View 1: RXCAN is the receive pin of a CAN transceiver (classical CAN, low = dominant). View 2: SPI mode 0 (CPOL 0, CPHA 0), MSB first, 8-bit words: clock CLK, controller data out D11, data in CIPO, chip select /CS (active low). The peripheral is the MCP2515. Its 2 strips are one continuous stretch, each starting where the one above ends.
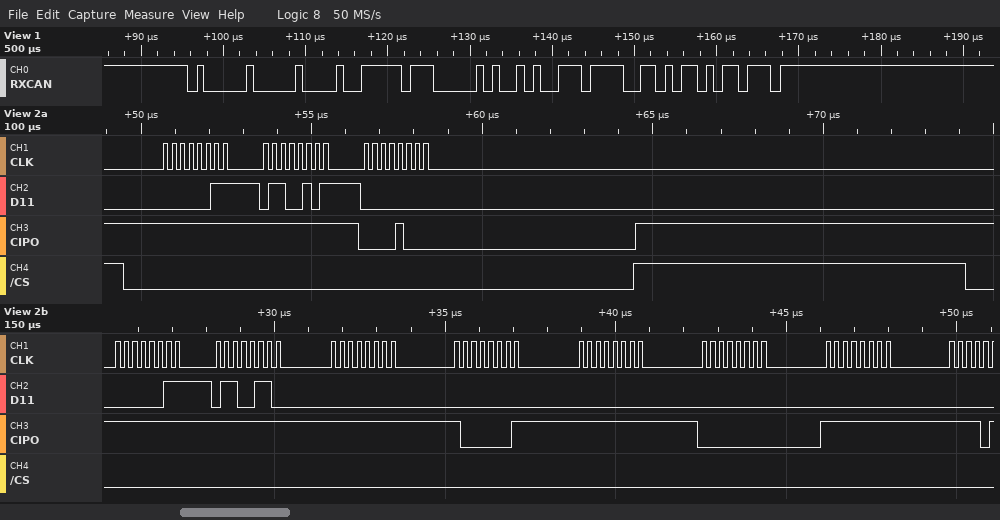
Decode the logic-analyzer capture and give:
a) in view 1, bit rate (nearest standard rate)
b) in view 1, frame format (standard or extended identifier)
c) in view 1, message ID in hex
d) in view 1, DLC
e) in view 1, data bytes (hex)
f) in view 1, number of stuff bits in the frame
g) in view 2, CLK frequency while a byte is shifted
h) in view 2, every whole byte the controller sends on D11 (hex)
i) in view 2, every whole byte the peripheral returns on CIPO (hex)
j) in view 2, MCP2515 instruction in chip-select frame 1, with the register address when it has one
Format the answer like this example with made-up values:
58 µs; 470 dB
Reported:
1000 kbit/s; standard; 0x400; 4; FF 02 53 BC; 4; 4 MHz; 0x03 0x65 0x00 0x03 0x66 0x00 0x00 0x00 0x00 0x00; 0xFF 0xFF 0x08 0xFF 0xFF 0xFF 0x81 0xFF 0x00 0xFF; READ 0x65
